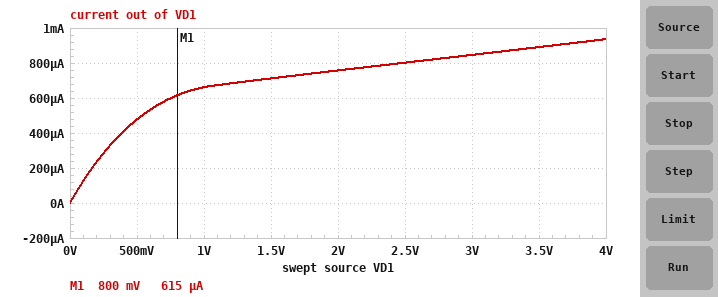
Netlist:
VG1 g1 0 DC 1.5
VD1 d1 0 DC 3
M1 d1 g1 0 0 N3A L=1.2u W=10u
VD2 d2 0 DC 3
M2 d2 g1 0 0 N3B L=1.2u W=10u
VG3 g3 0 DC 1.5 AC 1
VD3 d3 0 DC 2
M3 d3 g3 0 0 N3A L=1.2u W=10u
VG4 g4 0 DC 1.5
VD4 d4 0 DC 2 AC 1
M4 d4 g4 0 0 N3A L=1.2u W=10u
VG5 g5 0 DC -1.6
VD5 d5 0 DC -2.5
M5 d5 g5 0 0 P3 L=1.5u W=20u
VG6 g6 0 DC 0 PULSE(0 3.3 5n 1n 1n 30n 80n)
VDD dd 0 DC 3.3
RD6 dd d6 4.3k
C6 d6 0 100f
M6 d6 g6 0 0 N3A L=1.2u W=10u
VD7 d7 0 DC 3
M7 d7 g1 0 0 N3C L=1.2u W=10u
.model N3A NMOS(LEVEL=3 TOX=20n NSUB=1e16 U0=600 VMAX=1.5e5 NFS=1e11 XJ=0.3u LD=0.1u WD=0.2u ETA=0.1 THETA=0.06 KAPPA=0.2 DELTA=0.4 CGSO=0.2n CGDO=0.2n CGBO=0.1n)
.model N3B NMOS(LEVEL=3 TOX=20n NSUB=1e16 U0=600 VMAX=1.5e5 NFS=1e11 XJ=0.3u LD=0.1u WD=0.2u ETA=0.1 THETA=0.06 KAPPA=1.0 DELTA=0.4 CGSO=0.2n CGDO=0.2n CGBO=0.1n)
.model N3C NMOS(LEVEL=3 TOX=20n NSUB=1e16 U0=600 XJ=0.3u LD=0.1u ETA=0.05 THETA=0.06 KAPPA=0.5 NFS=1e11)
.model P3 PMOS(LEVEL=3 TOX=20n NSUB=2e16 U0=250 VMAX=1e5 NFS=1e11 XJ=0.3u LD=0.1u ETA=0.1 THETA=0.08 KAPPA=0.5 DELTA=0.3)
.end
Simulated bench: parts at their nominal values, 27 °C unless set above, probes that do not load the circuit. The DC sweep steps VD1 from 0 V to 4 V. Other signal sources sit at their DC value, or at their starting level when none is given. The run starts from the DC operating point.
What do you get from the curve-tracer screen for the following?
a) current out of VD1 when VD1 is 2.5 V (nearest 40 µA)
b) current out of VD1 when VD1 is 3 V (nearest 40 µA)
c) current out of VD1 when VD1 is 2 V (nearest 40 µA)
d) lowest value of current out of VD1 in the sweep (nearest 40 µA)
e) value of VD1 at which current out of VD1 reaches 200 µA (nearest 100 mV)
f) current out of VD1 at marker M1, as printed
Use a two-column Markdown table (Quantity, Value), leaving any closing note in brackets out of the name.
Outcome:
| Quantity | Value |
|---|---|
| current out of VD1 when VD1 is 2.5 V | 800 µA |
| current out of VD1 when VD1 is 3 V | 840 µA |
| current out of VD1 when VD1 is 2 V | 760 µA |
| lowest value of current out of VD1 in the sweep | 0 A |
| value of VD1 at which current out of VD1 reaches 200 µA | 200 mV |
| current out of VD1 at marker M1, as printed | 615 µA |
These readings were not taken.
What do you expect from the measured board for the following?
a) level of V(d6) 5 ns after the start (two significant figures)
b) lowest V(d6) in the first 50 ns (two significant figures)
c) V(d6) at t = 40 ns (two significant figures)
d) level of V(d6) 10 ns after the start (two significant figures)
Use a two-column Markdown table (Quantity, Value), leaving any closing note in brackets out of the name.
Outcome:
| Quantity | Value |
|---|---|
| level of V(d6) 5 ns after the start | 3.3 V |
| lowest V(d6) in the first 50 ns | 290 mV |
| V(d6) at t = 40 ns | 3.3 V |
| level of V(d6) 10 ns after the start | 290 mV |
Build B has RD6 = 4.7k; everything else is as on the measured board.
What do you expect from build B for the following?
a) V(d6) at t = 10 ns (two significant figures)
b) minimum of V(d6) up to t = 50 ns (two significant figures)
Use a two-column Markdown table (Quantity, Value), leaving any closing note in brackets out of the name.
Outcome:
| Quantity | Value |
|---|---|
| V(d6) at t = 10 ns | 270 mV |
| minimum of V(d6) up to t = 50 ns | 260 mV |
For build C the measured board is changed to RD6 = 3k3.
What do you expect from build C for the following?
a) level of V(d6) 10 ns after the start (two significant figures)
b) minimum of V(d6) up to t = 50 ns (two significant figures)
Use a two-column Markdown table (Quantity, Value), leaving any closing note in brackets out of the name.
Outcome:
| Quantity | Value |
|---|---|
| level of V(d6) 10 ns after the start | 390 mV |
| minimum of V(d6) up to t = 50 ns | 380 mV |
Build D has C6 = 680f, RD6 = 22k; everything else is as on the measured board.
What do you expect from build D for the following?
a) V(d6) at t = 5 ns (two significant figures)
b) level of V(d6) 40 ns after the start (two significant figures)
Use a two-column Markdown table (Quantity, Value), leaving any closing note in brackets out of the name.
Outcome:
| Quantity | Value |
|---|---|
| V(d6) at t = 5 ns | 3.1 V |
| level of V(d6) 40 ns after the start | 690 mV |
